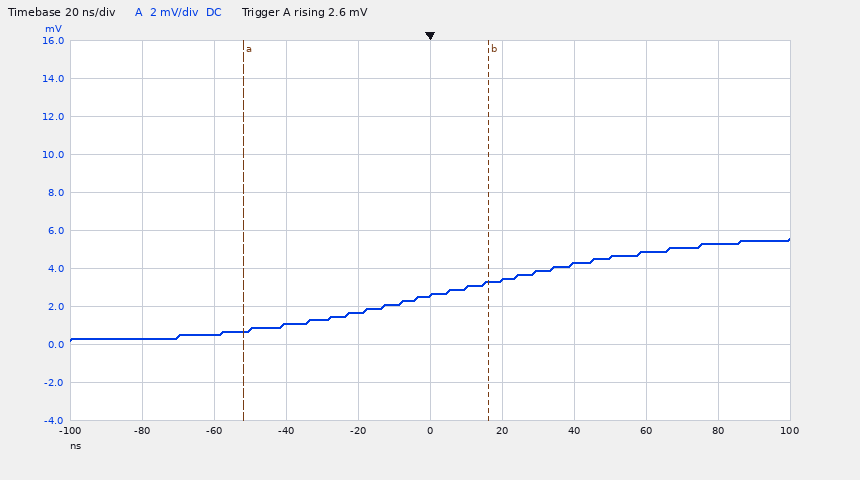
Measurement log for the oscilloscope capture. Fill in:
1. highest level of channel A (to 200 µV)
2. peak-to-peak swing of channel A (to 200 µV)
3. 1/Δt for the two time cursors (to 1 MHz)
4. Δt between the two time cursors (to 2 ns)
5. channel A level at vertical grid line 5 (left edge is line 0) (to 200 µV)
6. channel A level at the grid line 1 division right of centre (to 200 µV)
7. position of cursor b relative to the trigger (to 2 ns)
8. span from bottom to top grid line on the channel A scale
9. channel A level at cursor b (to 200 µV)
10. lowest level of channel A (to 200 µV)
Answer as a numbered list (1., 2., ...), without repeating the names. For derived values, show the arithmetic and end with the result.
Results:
1. 5.6 mV
2. 5.6 mV − (200 µV) = 5.4 mV
3. 1 / 68 ns ≈ 15 MHz
4. 68 ns
5. 2.6 mV
6. 3.4 mV
7. +16 ns
8. 20 mV
9. 3.2 mV
10. 200 µV
